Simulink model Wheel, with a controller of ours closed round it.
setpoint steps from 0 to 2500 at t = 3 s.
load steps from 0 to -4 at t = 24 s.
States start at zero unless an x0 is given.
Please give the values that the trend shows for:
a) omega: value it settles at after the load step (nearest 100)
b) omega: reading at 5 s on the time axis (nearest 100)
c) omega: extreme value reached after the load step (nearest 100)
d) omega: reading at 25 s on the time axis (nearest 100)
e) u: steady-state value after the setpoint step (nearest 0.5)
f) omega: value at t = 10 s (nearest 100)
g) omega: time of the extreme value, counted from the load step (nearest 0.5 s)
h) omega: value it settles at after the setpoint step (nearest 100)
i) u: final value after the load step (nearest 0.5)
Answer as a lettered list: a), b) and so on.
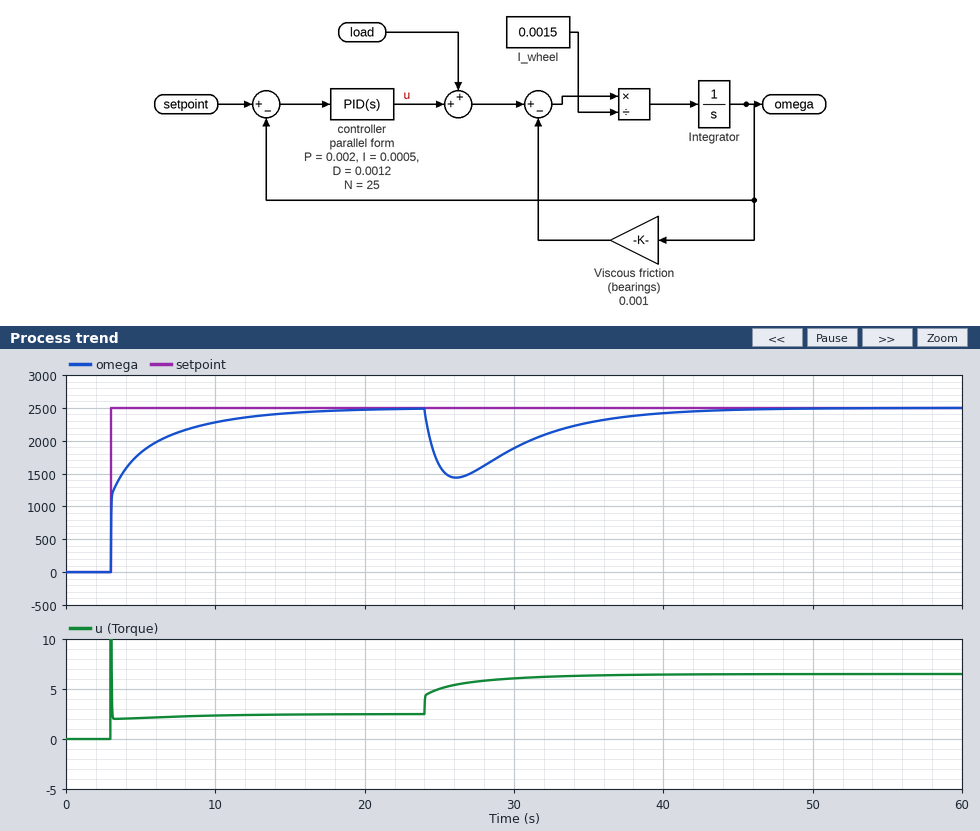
a) 2500
b) 1800
c) 1400
d) 1600
e) 2.5
f) 2300
g) 2.0 s
h) 2500
i) 6.5
